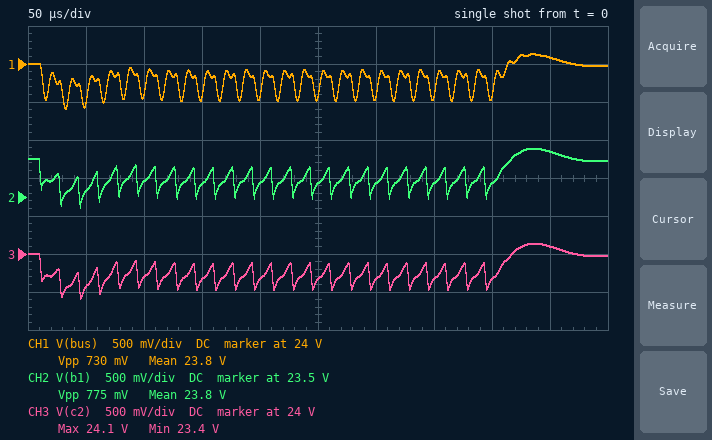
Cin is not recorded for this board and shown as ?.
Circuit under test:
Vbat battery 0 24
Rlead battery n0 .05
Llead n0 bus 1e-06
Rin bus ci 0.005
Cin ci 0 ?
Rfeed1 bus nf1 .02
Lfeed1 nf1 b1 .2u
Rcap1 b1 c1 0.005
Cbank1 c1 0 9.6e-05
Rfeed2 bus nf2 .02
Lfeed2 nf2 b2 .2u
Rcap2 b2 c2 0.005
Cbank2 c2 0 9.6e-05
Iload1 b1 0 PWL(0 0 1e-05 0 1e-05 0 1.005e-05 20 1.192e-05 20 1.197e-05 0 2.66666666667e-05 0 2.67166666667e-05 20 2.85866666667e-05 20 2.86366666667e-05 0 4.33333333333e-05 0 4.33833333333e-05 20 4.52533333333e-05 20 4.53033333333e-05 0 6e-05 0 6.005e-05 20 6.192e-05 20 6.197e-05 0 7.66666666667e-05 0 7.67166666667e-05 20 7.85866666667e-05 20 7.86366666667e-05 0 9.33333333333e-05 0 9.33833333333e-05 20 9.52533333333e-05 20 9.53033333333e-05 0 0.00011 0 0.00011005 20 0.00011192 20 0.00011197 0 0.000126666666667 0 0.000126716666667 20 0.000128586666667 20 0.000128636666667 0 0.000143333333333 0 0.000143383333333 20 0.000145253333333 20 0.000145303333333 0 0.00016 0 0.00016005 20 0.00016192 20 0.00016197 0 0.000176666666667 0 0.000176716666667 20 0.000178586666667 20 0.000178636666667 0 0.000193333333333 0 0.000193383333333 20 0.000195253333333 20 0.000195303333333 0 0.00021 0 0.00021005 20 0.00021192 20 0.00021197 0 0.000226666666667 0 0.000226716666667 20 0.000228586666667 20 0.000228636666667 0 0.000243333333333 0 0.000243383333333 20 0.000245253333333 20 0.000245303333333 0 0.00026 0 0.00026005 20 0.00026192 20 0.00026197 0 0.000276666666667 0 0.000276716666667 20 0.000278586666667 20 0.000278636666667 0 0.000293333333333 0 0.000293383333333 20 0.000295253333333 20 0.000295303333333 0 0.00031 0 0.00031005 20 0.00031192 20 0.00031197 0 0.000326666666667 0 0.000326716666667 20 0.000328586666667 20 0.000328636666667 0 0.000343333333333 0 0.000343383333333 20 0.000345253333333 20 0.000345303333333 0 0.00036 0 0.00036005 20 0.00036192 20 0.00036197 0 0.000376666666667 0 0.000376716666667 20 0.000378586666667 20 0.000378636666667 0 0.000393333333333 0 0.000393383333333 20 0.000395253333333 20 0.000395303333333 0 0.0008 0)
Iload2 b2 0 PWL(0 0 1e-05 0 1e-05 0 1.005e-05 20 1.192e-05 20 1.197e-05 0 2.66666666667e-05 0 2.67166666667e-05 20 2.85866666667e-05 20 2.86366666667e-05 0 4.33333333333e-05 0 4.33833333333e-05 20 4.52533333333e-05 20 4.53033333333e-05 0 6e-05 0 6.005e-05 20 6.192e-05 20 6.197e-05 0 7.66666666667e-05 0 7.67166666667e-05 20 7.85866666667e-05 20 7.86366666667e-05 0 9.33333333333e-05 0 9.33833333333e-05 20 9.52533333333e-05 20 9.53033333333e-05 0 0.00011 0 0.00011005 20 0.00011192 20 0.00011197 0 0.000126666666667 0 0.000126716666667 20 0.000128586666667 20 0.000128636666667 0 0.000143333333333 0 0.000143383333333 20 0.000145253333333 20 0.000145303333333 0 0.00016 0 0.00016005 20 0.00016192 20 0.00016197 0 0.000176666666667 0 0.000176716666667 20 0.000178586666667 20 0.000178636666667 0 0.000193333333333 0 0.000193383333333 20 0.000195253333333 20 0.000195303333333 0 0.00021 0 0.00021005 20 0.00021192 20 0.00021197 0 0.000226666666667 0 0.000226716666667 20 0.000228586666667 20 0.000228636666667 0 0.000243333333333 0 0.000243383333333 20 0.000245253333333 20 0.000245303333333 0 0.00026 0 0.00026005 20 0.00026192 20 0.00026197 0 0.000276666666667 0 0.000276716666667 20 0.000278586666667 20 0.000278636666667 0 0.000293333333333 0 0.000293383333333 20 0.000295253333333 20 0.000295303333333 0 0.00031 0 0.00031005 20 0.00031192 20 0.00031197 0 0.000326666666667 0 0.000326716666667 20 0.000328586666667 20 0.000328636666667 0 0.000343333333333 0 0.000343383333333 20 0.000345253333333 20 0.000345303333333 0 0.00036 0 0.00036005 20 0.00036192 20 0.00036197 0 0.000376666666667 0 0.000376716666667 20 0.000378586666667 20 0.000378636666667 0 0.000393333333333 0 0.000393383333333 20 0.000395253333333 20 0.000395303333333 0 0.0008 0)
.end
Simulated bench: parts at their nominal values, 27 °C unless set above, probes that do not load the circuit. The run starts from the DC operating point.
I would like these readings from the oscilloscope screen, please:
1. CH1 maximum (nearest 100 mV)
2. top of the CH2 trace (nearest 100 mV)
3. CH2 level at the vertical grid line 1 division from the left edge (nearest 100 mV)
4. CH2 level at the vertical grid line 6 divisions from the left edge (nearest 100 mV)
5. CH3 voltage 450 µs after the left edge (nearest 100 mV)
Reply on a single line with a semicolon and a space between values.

24.1 V; 24.1 V; 23.6 V; 23.7 V; 24.1 V
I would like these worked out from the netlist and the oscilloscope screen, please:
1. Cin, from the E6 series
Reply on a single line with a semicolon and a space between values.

33 µF
